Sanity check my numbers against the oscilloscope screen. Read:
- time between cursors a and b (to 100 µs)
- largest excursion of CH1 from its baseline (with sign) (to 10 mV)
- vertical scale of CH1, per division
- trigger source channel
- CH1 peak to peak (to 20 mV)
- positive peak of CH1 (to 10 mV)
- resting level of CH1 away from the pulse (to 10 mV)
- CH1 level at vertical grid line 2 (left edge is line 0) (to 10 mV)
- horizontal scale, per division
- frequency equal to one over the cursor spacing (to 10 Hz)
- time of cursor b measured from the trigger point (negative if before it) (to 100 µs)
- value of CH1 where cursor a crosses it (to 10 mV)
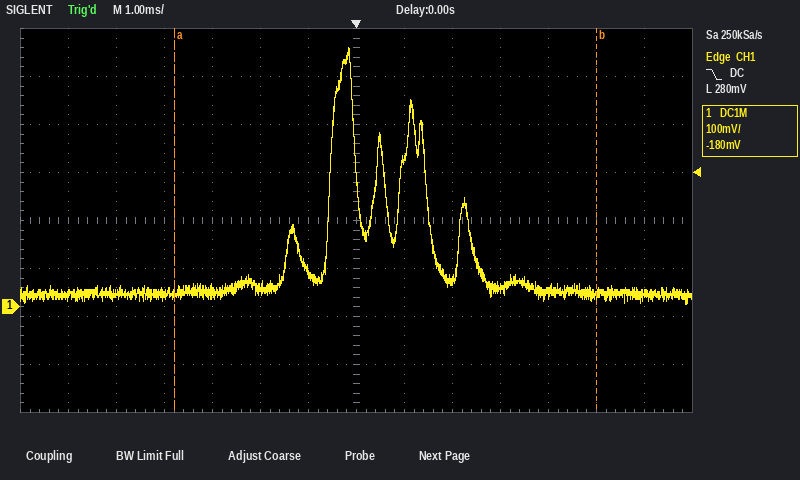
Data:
8.8 ms
+510 mV
100 mV
CH1
540 mV
540 mV
30 mV
30 mV
1 ms
110 Hz
+5.0 ms
30 mV
